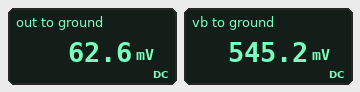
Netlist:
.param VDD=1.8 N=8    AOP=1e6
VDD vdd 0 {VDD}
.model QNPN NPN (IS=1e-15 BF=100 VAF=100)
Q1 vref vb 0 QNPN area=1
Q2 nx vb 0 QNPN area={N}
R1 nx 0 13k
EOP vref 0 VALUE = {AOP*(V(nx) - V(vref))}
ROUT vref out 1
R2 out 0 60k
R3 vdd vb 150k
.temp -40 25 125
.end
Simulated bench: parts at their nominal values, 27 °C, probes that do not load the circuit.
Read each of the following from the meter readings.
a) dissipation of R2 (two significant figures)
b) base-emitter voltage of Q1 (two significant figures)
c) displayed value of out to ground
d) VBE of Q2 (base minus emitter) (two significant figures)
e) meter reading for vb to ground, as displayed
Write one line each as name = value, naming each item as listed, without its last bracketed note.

dissipation of R2 = 65 nW
base-emitter voltage of Q1 = 550 mV
displayed value of out to ground = 62.6 mV
VBE of Q2 (base minus emitter) = 550 mV
meter reading for vb to ground, as displayed = 545.2 mV
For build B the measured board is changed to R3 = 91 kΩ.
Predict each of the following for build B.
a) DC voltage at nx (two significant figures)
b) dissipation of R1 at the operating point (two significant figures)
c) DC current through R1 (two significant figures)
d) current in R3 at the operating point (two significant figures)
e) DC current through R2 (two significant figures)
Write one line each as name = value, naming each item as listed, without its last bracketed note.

DC voltage at nx = 66 mV
dissipation of R1 at the operating point = 340 nW
DC current through R1 = 5.1 µA
current in R3 at the operating point = 14 µA
DC current through R2 = 1.1 µA
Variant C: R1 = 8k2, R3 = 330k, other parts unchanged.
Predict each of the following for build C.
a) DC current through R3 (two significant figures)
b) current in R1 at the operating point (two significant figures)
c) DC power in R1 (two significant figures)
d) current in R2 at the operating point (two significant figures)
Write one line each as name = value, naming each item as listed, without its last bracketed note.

DC current through R3 = 3.9 µA
current in R1 at the operating point = 5.2 µA
DC power in R1 = 220 nW
current in R2 at the operating point = 710 nA
